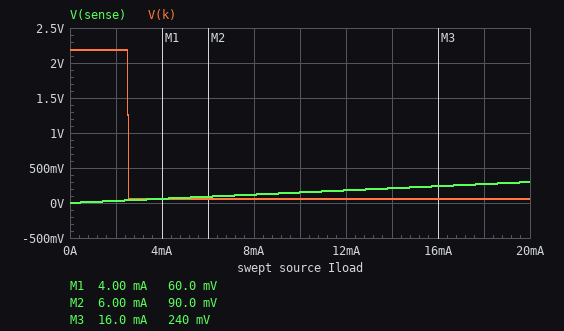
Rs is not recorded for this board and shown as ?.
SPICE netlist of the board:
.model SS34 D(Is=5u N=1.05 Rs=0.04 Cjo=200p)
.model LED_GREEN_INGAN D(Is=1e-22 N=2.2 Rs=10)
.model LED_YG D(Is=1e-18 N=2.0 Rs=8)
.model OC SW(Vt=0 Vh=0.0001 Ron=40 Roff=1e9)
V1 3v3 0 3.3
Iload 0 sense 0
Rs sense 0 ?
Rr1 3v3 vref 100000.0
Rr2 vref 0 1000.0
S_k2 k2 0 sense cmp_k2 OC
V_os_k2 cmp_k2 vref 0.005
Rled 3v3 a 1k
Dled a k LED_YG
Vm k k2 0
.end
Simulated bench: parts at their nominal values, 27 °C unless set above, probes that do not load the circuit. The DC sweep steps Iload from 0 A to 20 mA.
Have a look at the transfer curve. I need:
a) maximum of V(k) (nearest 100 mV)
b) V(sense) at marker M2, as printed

2.2 V
90.0 mV
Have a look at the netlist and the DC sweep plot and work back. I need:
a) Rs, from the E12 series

15 Ω
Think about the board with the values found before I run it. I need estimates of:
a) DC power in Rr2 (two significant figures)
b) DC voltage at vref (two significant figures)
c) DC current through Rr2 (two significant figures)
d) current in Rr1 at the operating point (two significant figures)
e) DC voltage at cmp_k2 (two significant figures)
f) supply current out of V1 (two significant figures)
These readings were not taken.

1.1 µW
33 mV
33 µA
33 µA
38 mV
33 µA
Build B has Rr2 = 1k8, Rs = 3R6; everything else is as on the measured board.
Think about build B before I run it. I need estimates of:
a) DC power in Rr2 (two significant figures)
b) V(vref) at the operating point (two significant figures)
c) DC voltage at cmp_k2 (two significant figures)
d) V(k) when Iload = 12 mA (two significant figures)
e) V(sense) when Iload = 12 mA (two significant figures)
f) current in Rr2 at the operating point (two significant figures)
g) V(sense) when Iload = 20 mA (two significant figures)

1.9 µW
58 mV
63 mV
2.2 V
43 mV
32 µA
72 mV
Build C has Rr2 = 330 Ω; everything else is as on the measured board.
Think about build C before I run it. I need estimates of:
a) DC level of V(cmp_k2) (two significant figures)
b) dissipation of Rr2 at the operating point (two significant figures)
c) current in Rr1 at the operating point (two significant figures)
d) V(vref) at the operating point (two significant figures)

16 mV
360 nW
33 µA
11 mV
